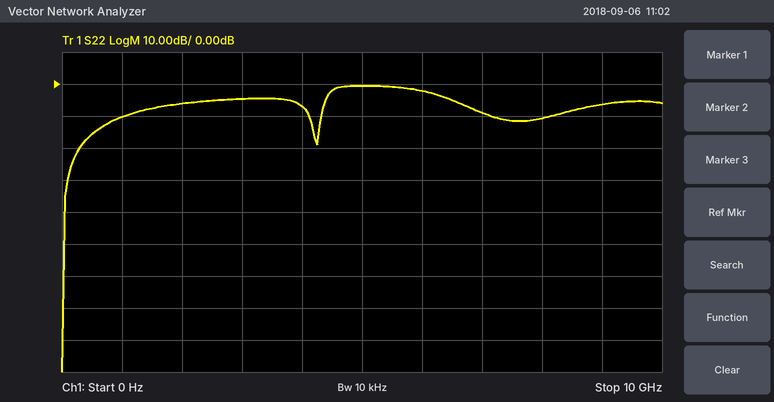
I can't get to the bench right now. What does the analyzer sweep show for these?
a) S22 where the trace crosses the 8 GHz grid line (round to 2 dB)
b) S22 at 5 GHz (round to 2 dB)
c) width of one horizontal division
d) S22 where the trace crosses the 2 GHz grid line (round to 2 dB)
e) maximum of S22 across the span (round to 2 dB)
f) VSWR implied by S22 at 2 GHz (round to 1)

-10 dB
0 dB
1 GHz
-6 dB
0 dB
3
